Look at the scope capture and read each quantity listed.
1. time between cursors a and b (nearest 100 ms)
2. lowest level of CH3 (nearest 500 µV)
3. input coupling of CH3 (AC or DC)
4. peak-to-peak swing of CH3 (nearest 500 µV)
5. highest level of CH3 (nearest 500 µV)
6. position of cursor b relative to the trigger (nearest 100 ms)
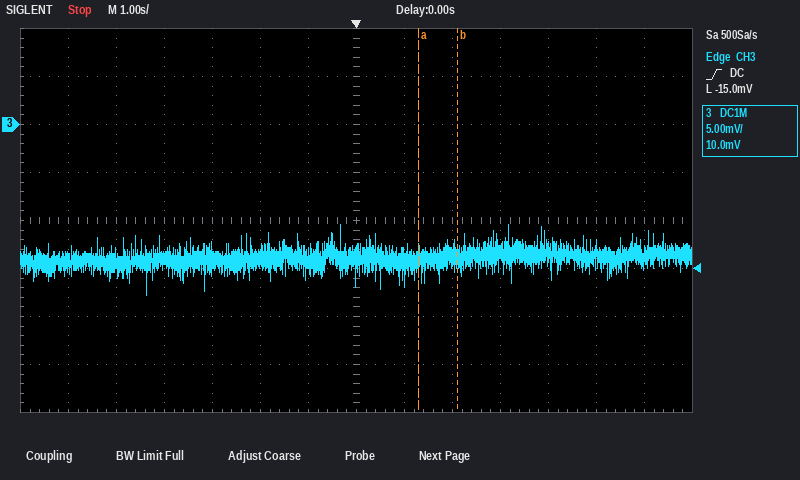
800 ms
-18.0 mV
DC
7.5 mV
-10.5 mV
+2.1 s
